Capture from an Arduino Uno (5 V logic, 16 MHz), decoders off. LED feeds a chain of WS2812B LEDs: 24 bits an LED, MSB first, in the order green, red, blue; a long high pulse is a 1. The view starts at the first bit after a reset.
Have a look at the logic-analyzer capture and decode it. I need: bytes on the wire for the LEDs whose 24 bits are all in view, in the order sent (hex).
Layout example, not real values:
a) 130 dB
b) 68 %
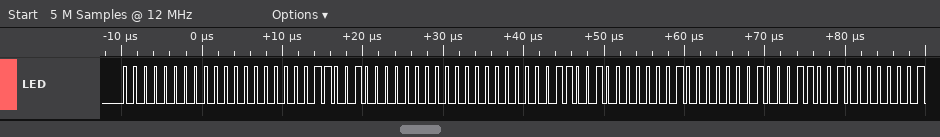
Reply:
a) 00 00 19 00 00 19 01 01 19
